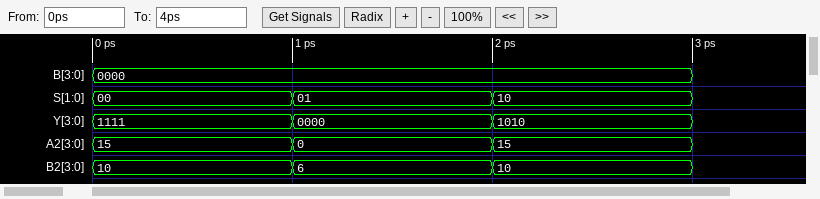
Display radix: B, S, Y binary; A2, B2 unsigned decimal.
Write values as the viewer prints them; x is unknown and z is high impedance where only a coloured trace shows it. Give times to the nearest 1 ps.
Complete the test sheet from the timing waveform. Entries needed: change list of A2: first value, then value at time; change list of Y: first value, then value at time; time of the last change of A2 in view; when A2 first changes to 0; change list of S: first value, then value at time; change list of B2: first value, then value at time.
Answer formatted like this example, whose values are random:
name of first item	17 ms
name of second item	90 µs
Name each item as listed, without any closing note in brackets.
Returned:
change list of A2: first value, then value at time	15, 0 at 1 ps, 15 at 2 ps
change list of Y: first value, then value at time	1111, 0000 at 1 ps, 1010 at 2 ps
time of the last change of A2 in view	2 ps
when A2 first changes to 0	1 ps
change list of S: first value, then value at time	00, 01 at 1 ps, 10 at 2 ps
change list of B2: first value, then value at time	10, 6 at 1 ps, 10 at 2 ps
